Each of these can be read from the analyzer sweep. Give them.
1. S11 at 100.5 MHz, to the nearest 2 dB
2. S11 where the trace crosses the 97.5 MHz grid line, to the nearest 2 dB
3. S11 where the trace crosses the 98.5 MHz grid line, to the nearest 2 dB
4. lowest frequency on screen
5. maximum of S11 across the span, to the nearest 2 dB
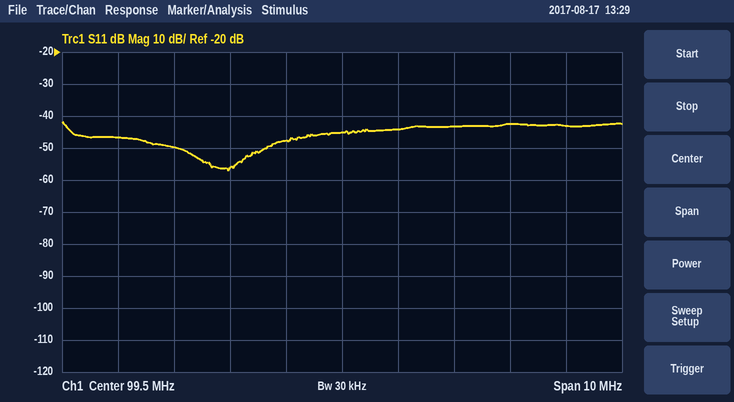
-44 dB
-56 dB
-48 dB
94.5 MHz
-42 dB
